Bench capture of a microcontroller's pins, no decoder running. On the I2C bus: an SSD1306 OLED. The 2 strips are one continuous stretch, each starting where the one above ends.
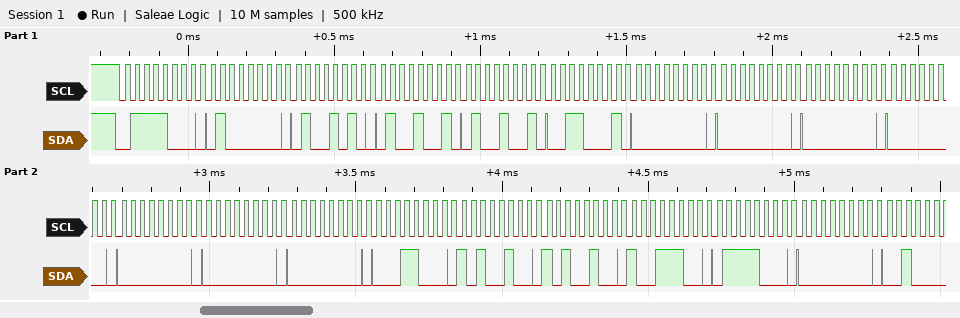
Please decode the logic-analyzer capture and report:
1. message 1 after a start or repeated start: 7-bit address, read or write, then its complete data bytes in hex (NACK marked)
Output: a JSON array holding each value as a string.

["0x3C write: 40 4A 49 49 31 00 00 00 00 00 00 00 18 A4 A4 9C 78 00"]
